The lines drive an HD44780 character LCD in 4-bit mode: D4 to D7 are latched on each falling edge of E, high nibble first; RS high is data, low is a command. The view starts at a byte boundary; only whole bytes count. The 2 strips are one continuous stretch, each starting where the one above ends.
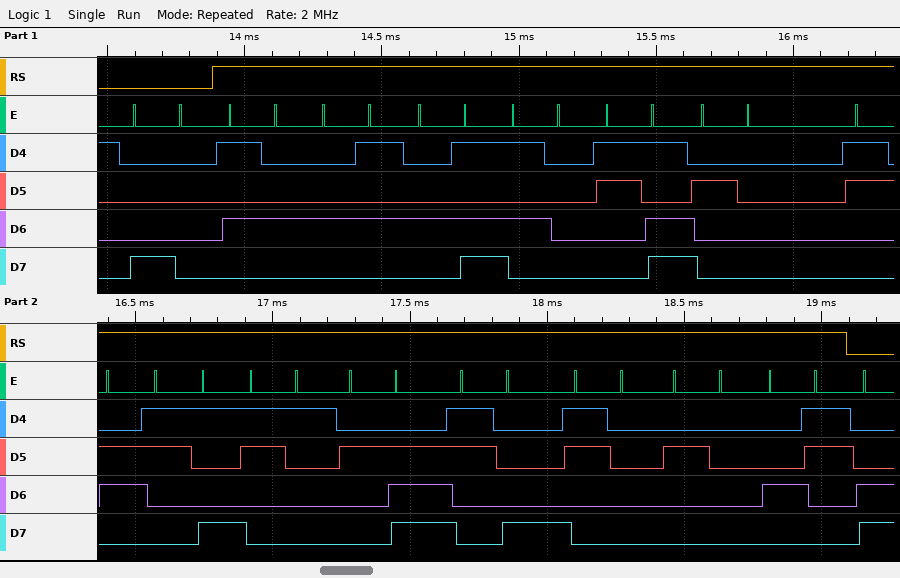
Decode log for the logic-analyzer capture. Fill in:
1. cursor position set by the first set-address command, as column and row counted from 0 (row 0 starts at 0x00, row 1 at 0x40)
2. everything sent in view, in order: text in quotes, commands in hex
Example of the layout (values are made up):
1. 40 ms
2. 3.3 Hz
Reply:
1. column 0, row 0
2. 0x80 "TEMP= 691.80 C"
